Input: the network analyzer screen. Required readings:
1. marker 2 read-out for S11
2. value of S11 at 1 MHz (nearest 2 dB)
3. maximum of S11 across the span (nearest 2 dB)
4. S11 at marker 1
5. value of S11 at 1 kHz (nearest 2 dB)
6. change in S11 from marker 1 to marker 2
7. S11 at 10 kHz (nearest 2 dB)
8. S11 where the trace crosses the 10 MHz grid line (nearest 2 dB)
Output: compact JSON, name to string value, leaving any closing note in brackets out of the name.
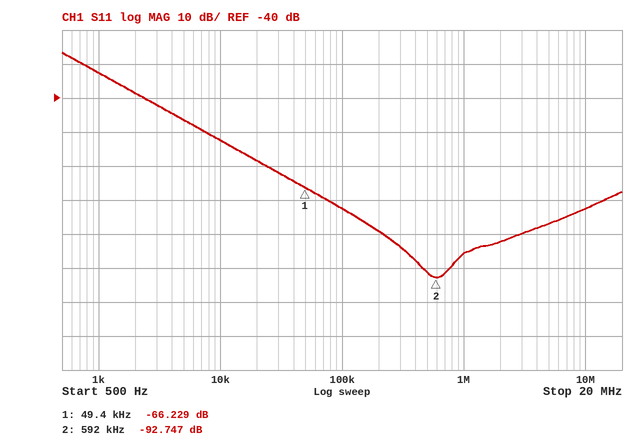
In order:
{"marker 2 read-out for S11": "-92.747 dB", "value of S11 at 1 MHz": "-86 dB", "maximum of S11 across the span": "-26 dB", "S11 at marker 1": "-66.229 dB", "value of S11 at 1 kHz": "-32 dB", "change in S11 from marker 1 to marker 2": "-26.518 dB", "S11 at 10 kHz": "-52 dB", "S11 where the trace crosses the 10 MHz grid line": "-72 dB"}
